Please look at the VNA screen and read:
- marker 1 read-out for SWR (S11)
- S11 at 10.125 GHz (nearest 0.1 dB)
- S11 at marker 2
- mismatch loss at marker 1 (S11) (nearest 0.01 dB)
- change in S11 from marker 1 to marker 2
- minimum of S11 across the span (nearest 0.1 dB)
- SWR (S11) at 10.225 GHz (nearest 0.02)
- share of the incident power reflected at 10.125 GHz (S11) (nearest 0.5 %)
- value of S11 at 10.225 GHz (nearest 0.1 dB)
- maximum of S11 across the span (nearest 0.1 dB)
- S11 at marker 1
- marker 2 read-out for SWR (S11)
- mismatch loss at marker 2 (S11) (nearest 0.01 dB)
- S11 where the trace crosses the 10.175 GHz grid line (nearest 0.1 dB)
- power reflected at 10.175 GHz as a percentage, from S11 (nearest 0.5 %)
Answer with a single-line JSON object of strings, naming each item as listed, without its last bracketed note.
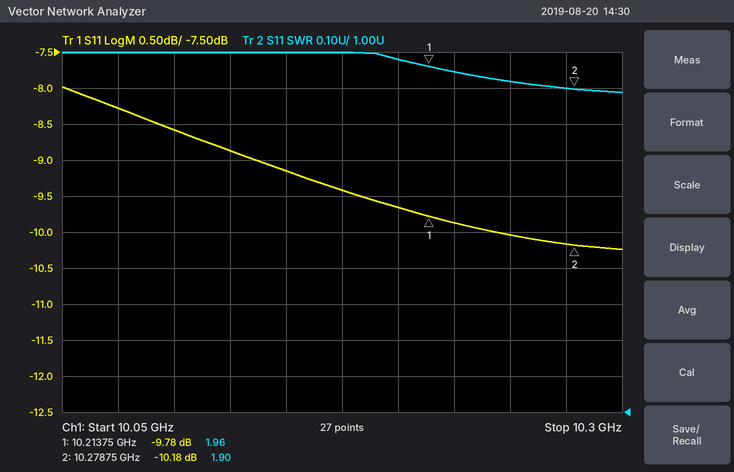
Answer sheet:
{"marker 1 read-out for SWR": "1.96", "S11 at 10.125 GHz": "-8.9 dB", "S11 at marker 2": "-10.18 dB", "mismatch loss at marker 1 (S11)": "0.48 dB", "change in S11 from marker 1 to marker 2": "-0.40 dB", "minimum of S11 across the span": "-10.2 dB", "SWR (S11) at 10.225 GHz": "1.94", "share of the incident power reflected at 10.125 GHz (S11)": "13.0 %", "value of S11 at 10.225 GHz": "-9.9 dB", "maximum of S11 across the span": "-8.0 dB", "S11 at marker 1": "-9.78 dB", "marker 2 read-out for SWR": "1.90", "mismatch loss at marker 2 (S11)": "0.44 dB", "S11 where the trace crosses the 10.175 GHz grid line": "-9.4 dB", "power reflected at 10.175 GHz as a percentage, from S11": "11.5 %"}
